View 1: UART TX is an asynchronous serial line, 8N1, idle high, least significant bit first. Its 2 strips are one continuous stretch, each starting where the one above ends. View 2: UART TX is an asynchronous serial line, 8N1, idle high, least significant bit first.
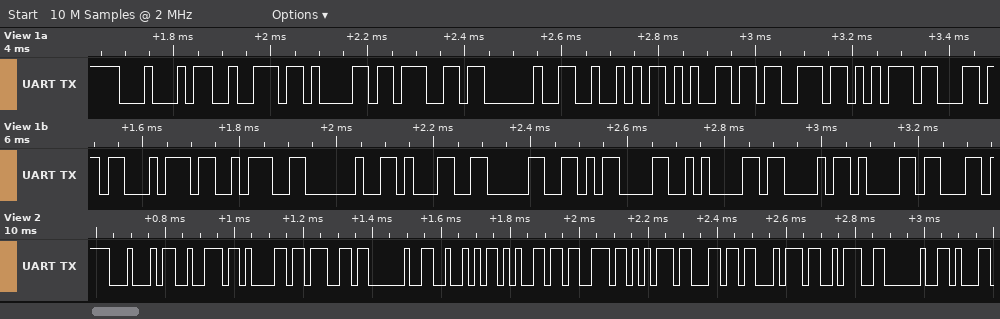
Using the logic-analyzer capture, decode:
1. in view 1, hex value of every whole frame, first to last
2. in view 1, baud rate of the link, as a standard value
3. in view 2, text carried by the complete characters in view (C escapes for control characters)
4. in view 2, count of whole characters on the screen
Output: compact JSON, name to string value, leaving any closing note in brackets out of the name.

{"in view 1, hex value of every whole frame, first to last": "44 72 61 67 20 52 65 73 75 6C 74 3A 20 31 30 0D 0A 43 61", "in view 1, baud rate of the link, as a standard value": "57600 baud", "in view 2, text carried by the complete characters in view": "\"Drag Result: \"", "in view 2, count of whole characters on the screen": "13"}
